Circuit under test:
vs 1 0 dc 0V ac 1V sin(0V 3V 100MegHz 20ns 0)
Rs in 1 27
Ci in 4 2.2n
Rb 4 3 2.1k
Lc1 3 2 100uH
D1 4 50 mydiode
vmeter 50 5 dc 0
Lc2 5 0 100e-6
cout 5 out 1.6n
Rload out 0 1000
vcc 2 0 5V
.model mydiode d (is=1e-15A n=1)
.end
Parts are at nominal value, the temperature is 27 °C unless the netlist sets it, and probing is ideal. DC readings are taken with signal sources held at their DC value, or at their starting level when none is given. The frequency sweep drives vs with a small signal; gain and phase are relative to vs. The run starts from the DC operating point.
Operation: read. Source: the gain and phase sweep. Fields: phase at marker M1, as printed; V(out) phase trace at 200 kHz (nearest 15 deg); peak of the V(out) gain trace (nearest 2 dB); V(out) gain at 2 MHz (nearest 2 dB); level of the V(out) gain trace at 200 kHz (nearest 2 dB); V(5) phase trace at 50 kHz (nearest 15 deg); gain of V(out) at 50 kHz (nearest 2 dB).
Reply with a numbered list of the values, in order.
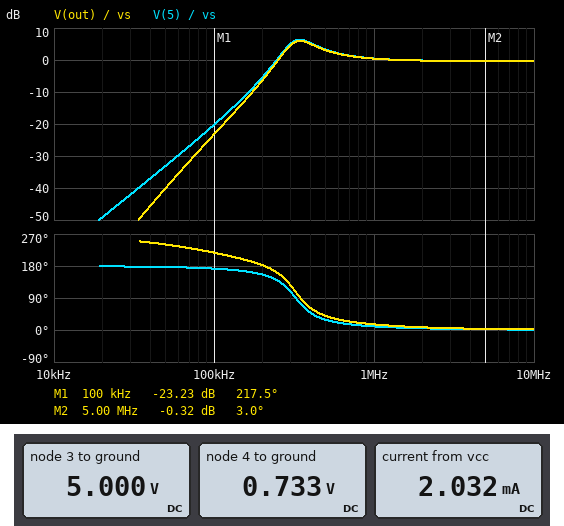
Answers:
1. 217.5 deg
2. 180 deg
3. 6 dB
4. 0 dB
5. -6 dB
6. 180 deg
7. -40 dB
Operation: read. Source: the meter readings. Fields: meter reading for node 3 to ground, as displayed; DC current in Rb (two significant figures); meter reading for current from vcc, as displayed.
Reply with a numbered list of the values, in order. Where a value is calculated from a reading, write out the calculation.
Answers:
1. 5.000 V
2. (5 V - 733 mV) / 2.1 kΩ = 2.0 mA
3. 2.032 mA
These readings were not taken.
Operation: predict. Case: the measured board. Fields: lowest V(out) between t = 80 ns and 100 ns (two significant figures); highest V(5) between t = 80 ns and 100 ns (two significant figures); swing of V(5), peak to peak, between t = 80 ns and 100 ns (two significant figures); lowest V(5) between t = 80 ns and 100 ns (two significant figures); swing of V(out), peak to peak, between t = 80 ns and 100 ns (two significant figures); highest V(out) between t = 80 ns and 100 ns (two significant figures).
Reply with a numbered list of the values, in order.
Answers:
1. -2.2 V
2. 2.9 V
3. 5.1 V
4. -2.2 V
5. 5.1 V
6. 2.9 V
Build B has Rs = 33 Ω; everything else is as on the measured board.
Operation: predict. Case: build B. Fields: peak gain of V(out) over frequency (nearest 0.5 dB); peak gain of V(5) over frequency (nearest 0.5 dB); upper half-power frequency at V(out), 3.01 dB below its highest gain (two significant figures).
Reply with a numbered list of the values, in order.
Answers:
1. 5.5 dB
2. 6.0 dB
3. 530 kHz
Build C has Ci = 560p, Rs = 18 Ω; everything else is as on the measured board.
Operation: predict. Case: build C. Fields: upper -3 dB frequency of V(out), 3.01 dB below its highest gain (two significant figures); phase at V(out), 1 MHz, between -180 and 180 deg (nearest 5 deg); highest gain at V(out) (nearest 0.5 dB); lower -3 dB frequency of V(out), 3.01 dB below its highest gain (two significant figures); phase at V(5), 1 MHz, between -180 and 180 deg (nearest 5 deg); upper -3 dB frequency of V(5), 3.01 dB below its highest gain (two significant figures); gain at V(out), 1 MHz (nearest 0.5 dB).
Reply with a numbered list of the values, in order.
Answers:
1. 2.1 MHz
2. 45 deg
3. 3.5 dB
4. 550 kHz
5. 40 deg
6. 2.0 MHz
7. 2.5 dB
